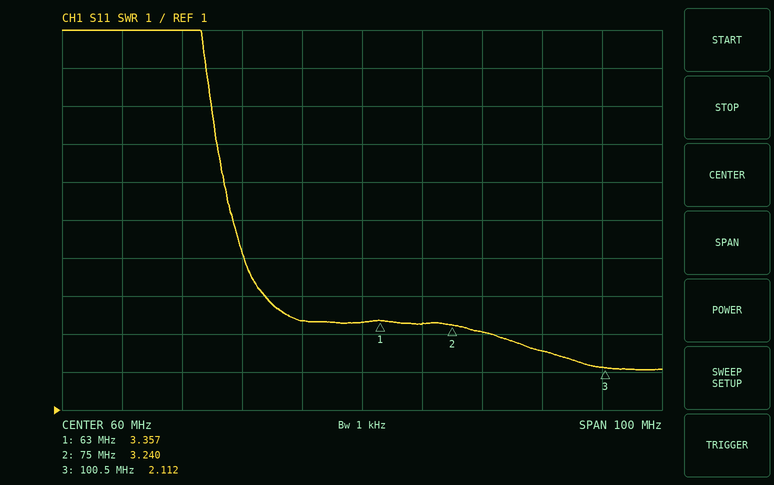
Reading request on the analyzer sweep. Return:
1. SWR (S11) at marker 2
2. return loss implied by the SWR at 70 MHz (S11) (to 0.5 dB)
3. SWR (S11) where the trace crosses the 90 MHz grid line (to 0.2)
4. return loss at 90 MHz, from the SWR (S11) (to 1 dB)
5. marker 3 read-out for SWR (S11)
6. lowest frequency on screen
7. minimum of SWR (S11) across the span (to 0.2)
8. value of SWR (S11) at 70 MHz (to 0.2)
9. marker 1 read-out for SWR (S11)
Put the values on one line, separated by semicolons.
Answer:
3.240; 5.5 dB; 2.6; 7 dB; 2.112; 10 MHz; 2.0; 3.2; 3.357
